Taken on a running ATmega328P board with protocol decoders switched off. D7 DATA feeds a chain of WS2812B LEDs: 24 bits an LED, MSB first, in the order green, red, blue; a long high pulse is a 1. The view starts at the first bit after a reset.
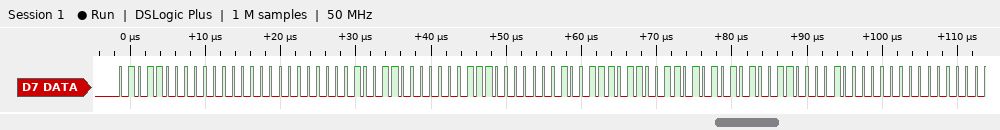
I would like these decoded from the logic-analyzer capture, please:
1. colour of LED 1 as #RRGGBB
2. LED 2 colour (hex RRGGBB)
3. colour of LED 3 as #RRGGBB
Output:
#005800
#074C01
#353B53
